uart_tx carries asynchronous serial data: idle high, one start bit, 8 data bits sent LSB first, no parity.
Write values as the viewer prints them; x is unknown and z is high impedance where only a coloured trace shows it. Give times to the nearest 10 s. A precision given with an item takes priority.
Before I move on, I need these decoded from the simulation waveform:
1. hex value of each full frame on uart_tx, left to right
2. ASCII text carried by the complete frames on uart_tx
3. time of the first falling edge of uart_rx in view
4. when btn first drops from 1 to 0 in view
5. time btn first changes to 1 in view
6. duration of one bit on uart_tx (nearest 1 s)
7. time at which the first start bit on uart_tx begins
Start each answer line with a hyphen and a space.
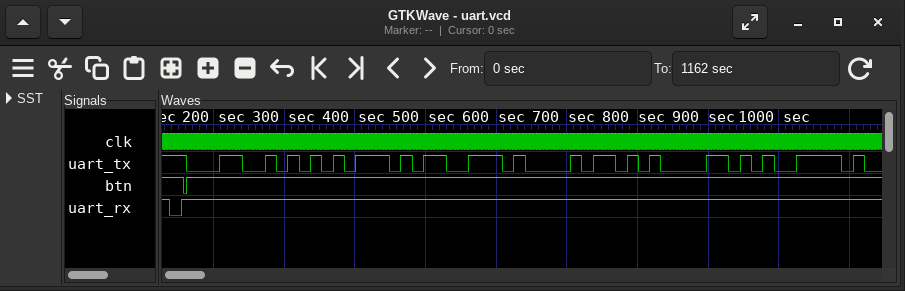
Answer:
- 4C, 75, 73, 68, 61, 79
- "Lushay"
- 140 s
- 160 s
- 160 s
- 16 s
- 160 s
